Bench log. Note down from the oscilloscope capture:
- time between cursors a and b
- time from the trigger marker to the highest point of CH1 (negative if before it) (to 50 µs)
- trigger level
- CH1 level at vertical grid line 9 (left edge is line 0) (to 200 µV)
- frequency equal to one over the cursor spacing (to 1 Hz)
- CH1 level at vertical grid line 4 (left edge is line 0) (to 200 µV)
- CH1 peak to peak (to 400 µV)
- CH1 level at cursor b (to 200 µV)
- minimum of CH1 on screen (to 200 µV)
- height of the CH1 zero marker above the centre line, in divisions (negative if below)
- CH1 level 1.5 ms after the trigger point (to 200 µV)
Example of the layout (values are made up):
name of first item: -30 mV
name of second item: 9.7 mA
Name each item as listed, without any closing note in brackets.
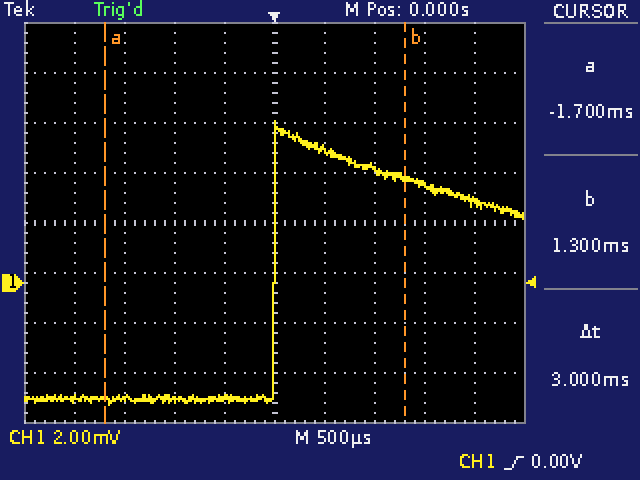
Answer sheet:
time between cursors a and b: 3 ms
time from the trigger marker to the highest point of CH1 (negative if before it): 0 µs
trigger level: 0.00 V
CH1 level at vertical grid line 9 (left edge is line 0): 3.2 mV
frequency equal to one over the cursor spacing: 333 Hz
CH1 level at vertical grid line 4 (left edge is line 0): -4.6 mV
CH1 peak to peak: 11.2 mV
CH1 level at cursor b: 4.2 mV
minimum of CH1 on screen: -4.8 mV
height of the CH1 zero marker above the centre line, in divisions: -1.2 div
CH1 level 1.5 ms after the trigger point: 4.0 mV
